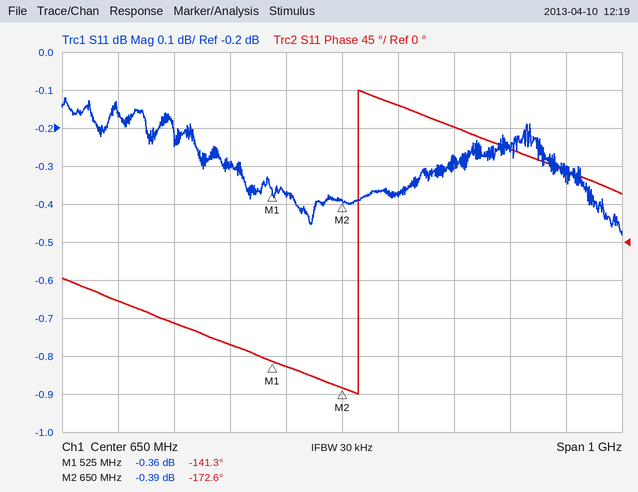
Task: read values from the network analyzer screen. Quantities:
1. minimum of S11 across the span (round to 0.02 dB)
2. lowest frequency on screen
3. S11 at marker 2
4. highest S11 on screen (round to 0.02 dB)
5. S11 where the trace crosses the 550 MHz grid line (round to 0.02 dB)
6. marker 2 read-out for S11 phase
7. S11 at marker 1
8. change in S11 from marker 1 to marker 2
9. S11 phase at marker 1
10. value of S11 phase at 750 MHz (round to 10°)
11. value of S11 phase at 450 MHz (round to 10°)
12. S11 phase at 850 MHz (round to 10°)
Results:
-0.48 dB
150 MHz
-0.39 dB
-0.12 dB
-0.38 dB
-172.6°
-0.36 dB
-0.03 dB
-141.3°
160°
-120°
140°
